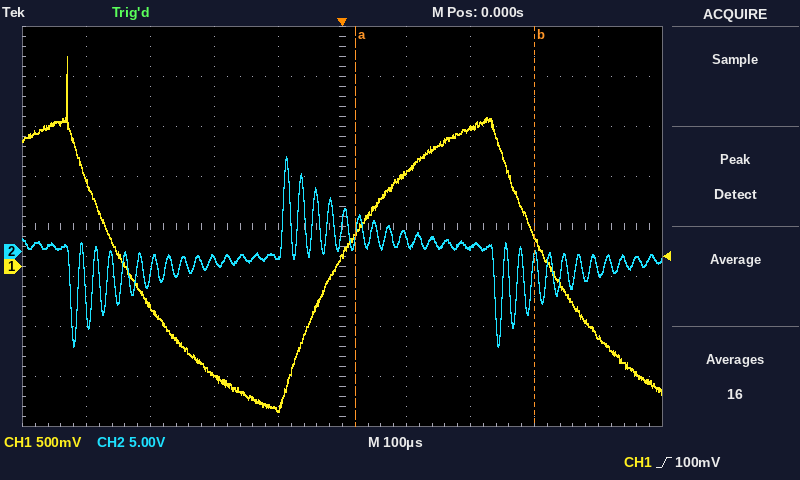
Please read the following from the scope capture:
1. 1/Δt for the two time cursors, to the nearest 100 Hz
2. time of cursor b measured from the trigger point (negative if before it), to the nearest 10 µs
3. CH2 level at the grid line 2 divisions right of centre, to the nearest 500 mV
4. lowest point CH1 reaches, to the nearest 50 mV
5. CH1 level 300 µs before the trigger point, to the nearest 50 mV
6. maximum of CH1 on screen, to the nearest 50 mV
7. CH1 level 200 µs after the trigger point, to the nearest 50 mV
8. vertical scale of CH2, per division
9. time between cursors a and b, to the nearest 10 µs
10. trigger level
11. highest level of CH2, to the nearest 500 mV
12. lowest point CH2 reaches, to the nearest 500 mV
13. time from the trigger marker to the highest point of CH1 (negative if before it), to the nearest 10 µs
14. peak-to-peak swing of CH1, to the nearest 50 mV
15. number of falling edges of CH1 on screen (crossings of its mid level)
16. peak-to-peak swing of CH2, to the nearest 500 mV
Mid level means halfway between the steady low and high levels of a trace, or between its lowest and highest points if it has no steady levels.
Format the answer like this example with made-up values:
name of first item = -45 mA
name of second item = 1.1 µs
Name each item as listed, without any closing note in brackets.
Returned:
1/Δt for the two time cursors, to the nearest 100 Hz = 3.6 kHz
time of cursor b measured from the trigger point (negative if before it), to the nearest 10 µs = +300 µs
CH2 level at the grid line 2 divisions right of centre, to the nearest 500 mV = 500 mV
lowest point CH1 reaches, to the nearest 50 mV = -1.45 V
CH1 level 300 µs before the trigger point, to the nearest 50 mV = -400 mV
maximum of CH1 on screen, to the nearest 50 mV = 2.10 V
CH1 level 200 µs after the trigger point, to the nearest 50 mV = 1.40 V
vertical scale of CH2, per division = 5 V
time between cursors a and b, to the nearest 10 µs = 280 µs
trigger level = 100 mV
highest level of CH2, to the nearest 500 mV = 9.5 V
lowest point CH2 reaches, to the nearest 500 mV = -9.5 V
time from the trigger marker to the highest point of CH1 (negative if before it), to the nearest 10 µs = -430 µs
peak-to-peak swing of CH1, to the nearest 50 mV = 3.55 V
number of falling edges of CH1 on screen = 2
peak-to-peak swing of CH2, to the nearest 500 mV = 19.0 V
